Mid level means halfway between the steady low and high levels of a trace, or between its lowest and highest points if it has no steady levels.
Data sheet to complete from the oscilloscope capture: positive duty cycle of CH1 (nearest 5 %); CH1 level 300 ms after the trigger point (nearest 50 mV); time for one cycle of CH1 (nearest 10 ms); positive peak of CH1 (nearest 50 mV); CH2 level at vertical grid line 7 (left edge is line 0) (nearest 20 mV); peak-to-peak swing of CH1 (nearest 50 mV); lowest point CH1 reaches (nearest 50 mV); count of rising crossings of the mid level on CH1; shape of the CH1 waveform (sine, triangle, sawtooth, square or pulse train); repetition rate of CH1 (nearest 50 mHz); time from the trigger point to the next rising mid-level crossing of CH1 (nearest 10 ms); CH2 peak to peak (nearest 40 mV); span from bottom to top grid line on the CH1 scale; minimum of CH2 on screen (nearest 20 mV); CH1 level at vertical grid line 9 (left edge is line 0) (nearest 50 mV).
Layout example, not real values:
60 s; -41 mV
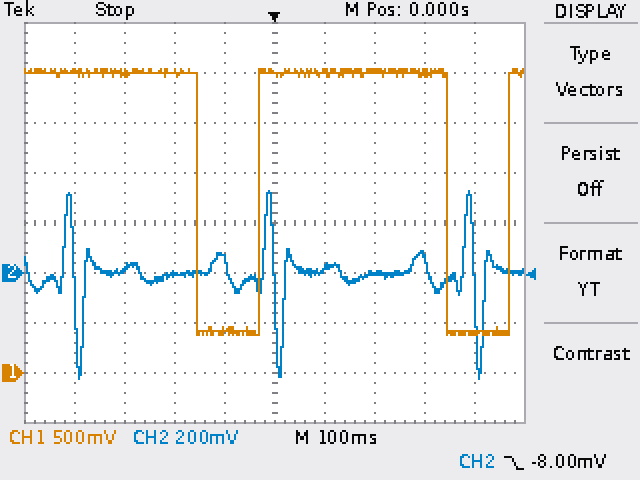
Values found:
75 %; 3.00 V; 500 ms; 3.05 V; 0 mV; 2.65 V; 400 mV; 2; pulse train; 2.00 Hz; 470 ms; 760 mV; 4 V; -420 mV; 400 mV
